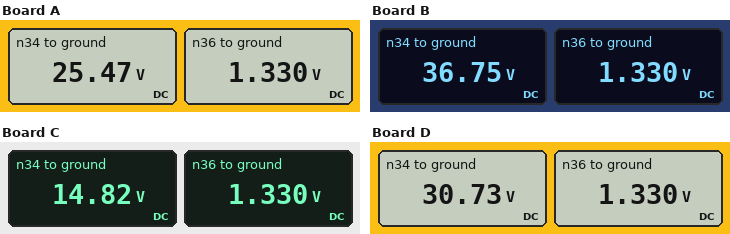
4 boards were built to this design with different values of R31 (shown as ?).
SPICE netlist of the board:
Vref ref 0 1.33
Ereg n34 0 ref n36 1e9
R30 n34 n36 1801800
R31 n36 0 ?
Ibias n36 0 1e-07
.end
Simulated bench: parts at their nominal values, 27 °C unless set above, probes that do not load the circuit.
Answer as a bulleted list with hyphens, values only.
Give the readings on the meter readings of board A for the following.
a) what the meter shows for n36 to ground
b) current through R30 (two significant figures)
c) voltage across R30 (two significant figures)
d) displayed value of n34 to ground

- 1.330 V
- 13 µA
- 24 V
- 25.47 V
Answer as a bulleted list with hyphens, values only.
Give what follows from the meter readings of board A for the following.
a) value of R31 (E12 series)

- 100 kΩ
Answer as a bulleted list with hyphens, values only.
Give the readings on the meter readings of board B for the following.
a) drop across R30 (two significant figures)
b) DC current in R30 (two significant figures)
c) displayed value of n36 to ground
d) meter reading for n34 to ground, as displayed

- 35 V
- 20 µA
- 1.330 V
- 36.75 V
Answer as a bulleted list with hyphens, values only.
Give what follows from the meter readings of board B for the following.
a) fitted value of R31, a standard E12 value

- 68 kΩ
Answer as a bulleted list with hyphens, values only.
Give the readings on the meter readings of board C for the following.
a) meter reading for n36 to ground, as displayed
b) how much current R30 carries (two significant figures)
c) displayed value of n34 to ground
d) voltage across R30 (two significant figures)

- 1.330 V
- 7.5 µA
- 14.82 V
- 13 V
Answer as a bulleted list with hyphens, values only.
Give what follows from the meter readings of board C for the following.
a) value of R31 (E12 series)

- 180 kΩ
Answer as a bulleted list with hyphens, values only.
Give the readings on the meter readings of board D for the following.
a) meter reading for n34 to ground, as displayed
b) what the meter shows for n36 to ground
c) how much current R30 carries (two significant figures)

- 30.73 V
- 1.330 V
- 16 µA
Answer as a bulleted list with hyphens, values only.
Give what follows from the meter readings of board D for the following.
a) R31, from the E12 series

- 82 kΩ
